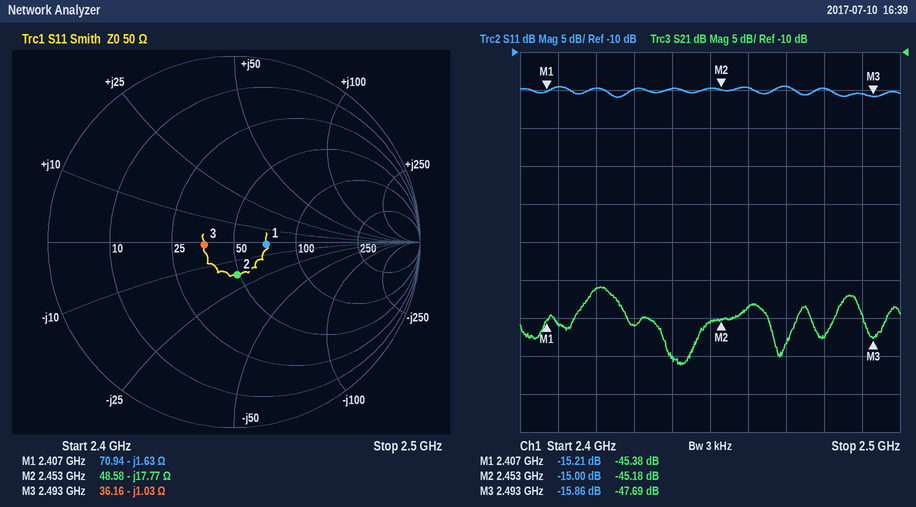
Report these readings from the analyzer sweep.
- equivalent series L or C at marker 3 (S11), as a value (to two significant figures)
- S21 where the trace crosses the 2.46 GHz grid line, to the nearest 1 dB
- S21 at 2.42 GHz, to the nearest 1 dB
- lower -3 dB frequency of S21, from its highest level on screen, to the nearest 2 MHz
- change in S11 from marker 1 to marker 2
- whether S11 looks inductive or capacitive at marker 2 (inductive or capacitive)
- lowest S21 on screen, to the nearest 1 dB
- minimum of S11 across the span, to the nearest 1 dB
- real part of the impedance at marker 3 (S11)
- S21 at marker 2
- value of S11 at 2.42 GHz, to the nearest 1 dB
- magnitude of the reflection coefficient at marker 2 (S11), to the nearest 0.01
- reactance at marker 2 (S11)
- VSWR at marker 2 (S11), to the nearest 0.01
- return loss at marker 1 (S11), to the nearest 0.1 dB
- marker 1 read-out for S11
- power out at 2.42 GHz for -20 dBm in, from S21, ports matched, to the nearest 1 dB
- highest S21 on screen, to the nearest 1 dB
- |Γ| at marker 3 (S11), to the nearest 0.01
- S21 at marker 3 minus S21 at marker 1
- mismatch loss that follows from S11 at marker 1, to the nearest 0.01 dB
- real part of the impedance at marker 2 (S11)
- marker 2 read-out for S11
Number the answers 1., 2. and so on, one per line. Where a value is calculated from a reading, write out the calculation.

1. C = 1/(2π × 2.493 GHz × 1.03 Ω) ≈ 62 pF
2. -44 dB
3. -41 dB
4. 2.416 GHz
5. -15 − (-15.21) = 0.21 dB
6. capacitive
7. -51 dB
8. -16 dB
9. 36.16 Ω
10. -45.18 dB
11. -15 dB
12. 10^(-15/20) ≈ 0.18
13. -17.77 Ω
14. 1.43
15. 15.2 dB
16. -15.21 dB
17. -20 dBm + (-41 dB) = -61 dBm
18. -41 dB
19. 0.16
20. -47.69 − (-45.38) = -2.31 dB
21. −10 log10(1 − 10^(-15.21/10)) ≈ 0.13 dB
22. 48.58 Ω
23. -15.00 dB
